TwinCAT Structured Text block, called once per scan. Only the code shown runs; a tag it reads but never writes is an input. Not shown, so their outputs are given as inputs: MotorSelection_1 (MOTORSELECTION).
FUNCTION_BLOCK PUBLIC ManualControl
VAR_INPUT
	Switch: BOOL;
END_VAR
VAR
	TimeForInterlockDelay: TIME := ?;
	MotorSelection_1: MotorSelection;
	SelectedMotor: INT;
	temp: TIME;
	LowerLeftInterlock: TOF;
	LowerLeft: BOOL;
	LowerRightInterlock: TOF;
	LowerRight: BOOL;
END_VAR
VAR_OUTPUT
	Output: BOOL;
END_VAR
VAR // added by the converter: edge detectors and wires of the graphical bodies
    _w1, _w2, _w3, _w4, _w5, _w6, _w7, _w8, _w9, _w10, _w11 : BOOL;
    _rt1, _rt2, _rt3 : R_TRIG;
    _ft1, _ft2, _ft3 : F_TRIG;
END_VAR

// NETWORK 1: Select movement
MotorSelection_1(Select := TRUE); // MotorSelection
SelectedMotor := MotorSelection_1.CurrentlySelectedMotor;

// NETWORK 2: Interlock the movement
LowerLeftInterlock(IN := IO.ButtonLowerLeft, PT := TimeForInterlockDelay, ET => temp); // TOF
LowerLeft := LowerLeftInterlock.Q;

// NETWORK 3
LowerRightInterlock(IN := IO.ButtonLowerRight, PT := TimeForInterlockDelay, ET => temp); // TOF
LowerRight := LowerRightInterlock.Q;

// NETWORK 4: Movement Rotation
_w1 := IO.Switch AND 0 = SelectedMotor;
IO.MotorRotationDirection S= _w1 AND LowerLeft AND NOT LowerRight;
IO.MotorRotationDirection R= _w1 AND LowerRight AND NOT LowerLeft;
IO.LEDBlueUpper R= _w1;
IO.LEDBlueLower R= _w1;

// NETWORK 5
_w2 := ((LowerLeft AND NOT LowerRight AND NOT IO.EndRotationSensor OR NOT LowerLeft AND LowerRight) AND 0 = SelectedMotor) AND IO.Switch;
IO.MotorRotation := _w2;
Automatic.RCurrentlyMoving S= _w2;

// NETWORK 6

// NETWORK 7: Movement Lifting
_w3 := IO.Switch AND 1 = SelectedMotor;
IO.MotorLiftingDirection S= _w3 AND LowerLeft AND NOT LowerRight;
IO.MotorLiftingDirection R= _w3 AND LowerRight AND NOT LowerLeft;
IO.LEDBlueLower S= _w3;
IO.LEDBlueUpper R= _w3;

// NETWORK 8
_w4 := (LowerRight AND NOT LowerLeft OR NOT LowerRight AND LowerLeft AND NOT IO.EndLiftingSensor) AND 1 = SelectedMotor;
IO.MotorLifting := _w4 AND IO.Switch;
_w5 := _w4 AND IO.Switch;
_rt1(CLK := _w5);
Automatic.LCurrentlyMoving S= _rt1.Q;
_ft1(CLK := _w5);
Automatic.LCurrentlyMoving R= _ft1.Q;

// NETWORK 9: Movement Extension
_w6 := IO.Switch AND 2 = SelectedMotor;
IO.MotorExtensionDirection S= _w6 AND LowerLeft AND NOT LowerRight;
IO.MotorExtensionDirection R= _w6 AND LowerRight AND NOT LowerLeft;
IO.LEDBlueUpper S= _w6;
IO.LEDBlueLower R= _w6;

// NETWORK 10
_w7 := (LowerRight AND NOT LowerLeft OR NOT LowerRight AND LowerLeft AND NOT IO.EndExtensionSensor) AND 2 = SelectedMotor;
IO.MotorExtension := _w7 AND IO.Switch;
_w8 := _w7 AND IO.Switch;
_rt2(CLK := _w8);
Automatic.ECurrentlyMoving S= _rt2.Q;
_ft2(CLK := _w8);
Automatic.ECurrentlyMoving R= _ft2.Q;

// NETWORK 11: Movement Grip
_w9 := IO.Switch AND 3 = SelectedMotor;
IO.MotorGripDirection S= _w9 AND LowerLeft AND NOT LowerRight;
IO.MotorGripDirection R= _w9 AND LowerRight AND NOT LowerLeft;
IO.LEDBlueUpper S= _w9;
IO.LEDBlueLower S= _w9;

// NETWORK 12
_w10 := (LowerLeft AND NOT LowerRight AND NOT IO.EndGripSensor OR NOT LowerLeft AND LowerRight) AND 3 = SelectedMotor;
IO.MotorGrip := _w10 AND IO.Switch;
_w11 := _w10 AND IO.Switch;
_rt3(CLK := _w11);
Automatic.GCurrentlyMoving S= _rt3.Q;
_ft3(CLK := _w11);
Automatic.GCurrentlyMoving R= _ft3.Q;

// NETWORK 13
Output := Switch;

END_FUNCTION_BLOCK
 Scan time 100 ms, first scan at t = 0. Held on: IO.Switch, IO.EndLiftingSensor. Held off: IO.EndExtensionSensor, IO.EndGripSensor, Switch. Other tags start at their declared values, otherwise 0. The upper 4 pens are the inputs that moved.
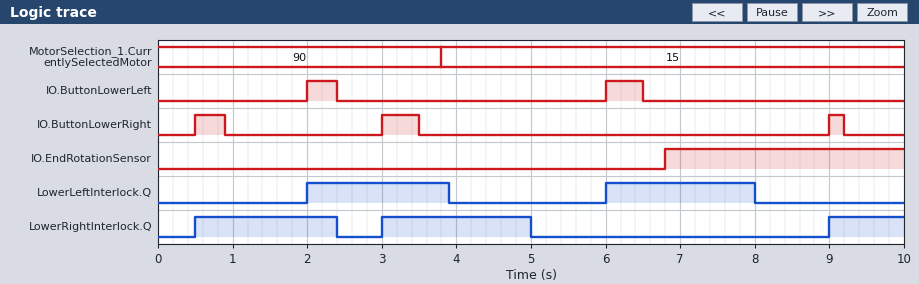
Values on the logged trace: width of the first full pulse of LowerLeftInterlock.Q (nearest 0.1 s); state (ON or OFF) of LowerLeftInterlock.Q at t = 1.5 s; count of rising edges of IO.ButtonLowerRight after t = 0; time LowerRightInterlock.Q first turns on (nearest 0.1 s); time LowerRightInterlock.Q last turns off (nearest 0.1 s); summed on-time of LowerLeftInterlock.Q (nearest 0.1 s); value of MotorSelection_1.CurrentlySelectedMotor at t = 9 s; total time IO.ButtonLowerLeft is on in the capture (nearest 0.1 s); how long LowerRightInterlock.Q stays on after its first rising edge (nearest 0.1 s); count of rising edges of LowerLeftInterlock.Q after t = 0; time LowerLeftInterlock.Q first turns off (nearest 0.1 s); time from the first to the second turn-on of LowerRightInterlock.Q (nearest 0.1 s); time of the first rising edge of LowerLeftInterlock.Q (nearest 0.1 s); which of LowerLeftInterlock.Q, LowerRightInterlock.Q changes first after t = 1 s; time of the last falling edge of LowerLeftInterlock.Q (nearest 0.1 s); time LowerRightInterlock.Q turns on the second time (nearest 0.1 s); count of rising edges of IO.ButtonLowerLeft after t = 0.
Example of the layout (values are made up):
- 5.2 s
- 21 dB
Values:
- 1.9 s
- OFF
- 3
- 0.5 s
- 5.0 s
- 3.9 s
- 15
- 0.9 s
- 1.9 s
- 2
- 3.9 s
- 2.5 s
- 2.0 s
- LowerLeftInterlock.Q
- 8.0 s
- 3.0 s
- 2
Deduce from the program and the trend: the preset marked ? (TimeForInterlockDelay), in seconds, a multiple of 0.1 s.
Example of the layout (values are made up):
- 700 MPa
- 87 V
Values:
- 1.5 s
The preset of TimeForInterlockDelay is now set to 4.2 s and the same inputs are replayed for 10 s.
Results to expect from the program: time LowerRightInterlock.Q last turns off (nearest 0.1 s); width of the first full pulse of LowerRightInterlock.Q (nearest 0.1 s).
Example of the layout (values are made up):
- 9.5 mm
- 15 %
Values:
- 7.7 s
- 7.2 s
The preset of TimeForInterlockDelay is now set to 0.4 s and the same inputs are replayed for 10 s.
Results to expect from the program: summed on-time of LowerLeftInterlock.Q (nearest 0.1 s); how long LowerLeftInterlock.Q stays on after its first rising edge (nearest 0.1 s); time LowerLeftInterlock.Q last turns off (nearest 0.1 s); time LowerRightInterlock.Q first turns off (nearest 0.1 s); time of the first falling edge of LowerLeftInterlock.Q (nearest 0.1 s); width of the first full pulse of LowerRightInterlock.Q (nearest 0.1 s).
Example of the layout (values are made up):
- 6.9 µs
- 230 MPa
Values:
- 1.7 s
- 0.8 s
- 6.9 s
- 1.3 s
- 2.8 s
- 0.8 s
